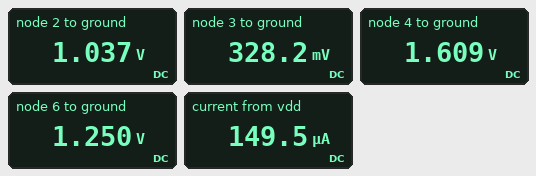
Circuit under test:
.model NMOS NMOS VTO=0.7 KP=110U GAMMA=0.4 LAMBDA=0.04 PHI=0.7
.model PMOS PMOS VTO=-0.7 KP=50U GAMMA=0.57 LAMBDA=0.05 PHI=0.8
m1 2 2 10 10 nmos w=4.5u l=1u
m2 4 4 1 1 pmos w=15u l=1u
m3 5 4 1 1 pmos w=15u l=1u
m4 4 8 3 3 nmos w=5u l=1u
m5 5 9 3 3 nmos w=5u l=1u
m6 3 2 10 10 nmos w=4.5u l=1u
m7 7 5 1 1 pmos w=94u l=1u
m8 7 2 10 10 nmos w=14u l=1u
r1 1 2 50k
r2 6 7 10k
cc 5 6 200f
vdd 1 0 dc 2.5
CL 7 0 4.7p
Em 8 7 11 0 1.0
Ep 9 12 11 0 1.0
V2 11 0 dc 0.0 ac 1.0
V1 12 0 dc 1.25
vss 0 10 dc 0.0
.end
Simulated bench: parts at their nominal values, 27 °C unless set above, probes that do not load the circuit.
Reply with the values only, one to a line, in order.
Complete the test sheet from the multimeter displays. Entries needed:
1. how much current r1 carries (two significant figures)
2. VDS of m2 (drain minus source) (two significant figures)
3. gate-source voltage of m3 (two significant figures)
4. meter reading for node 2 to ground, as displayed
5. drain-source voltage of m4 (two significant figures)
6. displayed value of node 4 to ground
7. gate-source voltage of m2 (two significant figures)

29 µA
-890 mV
-890 mV
1.037 V
1.3 V
1.609 V
-890 mV
